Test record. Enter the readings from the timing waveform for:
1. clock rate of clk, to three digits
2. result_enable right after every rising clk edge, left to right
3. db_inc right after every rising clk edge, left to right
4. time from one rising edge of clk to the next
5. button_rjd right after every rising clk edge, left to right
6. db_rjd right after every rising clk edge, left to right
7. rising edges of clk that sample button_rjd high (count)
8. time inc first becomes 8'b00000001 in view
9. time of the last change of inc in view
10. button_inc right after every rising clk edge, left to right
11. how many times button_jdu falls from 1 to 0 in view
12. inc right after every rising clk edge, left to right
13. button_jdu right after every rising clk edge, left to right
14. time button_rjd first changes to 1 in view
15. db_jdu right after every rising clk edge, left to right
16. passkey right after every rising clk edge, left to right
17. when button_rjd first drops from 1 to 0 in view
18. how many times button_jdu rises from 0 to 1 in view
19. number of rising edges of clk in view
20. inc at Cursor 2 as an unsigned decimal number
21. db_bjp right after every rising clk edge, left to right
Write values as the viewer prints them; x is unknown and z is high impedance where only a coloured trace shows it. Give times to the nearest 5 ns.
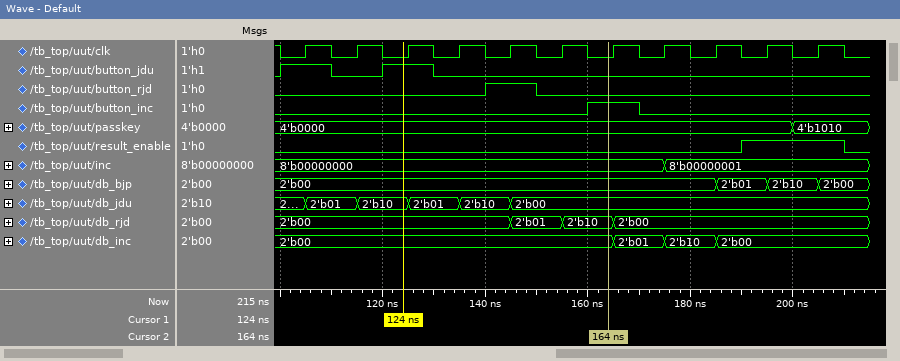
100 MHz
0 0 0 0 0 0 0 0 0 1 1
2'b00, 2'b00, 2'b00, 2'b00, 2'b00, 2'b00, 2'b01, 2'b10, 2'b00, 2'b00, 2'b00
10 ns
0 0 0 0 1 0 0 0 0 0 0
2'b00, 2'b00, 2'b00, 2'b00, 2'b01, 2'b10, 2'b00, 2'b00, 2'b00, 2'b00, 2'b00
1
175 ns
175 ns
0 0 0 0 0 0 1 0 0 0 0
2
8'b00000000, 8'b00000000, 8'b00000000, 8'b00000000, 8'b00000000, 8'b00000000, 8'b00000000, 8'b00000001, 8'b00000001, 8'b00000001, 8'b00000001
1 0 1 0 0 0 0 0 0 0 0
140 ns
2'b01, 2'b10, 2'b01, 2'b10, 2'b00, 2'b00, 2'b00, 2'b00, 2'b00, 2'b00, 2'b00
4'b0000, 4'b0000, 4'b0000, 4'b0000, 4'b0000, 4'b0000, 4'b0000, 4'b0000, 4'b0000, 4'b0000, 4'b1010
150 ns
2
11
0
2'b00, 2'b00, 2'b00, 2'b00, 2'b00, 2'b00, 2'b00, 2'b00, 2'b01, 2'b10, 2'b00
